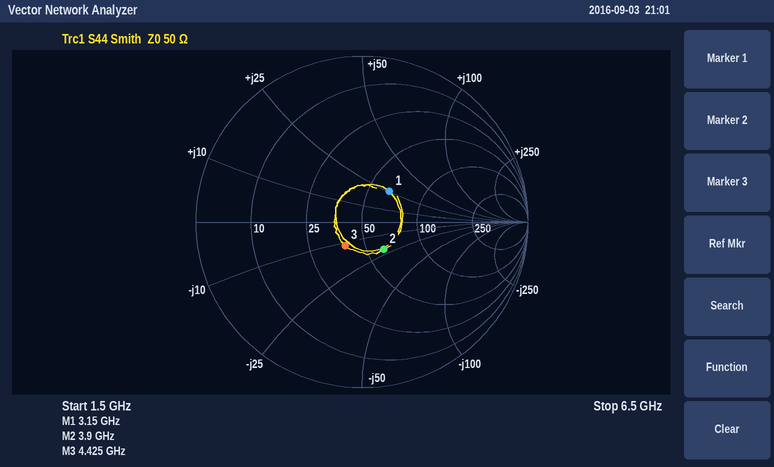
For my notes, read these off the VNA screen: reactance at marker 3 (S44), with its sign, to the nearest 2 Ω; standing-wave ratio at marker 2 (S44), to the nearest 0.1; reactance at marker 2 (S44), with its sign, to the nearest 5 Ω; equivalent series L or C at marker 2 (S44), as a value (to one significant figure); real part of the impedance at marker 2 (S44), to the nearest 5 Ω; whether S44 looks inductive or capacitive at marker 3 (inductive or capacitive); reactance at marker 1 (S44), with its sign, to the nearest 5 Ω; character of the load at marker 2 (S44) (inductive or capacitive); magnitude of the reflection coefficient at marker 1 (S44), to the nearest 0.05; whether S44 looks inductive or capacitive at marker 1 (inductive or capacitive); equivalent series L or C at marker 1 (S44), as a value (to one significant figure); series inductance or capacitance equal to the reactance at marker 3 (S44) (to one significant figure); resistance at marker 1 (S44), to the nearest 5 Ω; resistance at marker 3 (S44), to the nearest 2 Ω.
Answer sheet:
-12 Ω
1.5
-20 Ω
2 pF
60 Ω
capacitive
+25 Ω
capacitive
0.25
inductive
1 nH
3 pF
65 Ω
40 Ω
